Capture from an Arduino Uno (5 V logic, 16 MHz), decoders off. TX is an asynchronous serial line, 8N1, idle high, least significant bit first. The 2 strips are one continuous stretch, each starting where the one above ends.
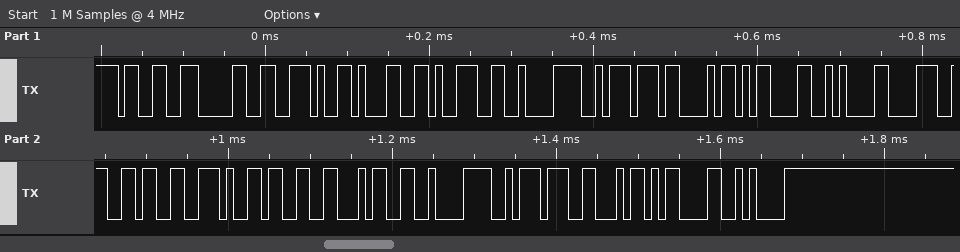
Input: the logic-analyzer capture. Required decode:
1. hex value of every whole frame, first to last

0x33 0x30 0x2E 0x31 0x39 0xC2 0xBA 0x43 0x0D 0x0A 0x38 0x36 0x2E 0x33 0x34 0xC2 0xBA 0x46 0x0D 0x0A
